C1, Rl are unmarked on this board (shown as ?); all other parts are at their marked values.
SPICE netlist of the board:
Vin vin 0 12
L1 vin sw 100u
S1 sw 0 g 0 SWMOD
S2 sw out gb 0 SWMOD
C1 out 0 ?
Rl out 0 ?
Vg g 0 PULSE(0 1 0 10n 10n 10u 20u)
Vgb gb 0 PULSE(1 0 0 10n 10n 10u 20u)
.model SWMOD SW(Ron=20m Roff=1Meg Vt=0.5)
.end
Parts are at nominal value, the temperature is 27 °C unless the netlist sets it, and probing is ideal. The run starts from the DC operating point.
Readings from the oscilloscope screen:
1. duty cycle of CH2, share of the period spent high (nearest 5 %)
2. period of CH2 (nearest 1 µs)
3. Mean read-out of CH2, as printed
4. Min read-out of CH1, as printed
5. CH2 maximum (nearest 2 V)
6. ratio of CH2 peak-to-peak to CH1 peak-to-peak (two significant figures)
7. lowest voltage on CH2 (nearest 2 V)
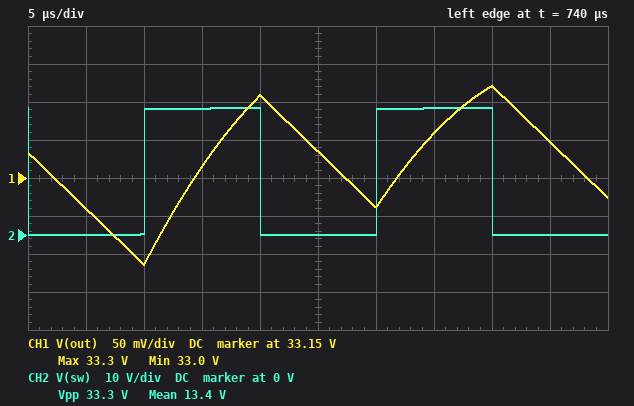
50 %
20 µs
13.4 V
33.0 V
34 V
140
0 V
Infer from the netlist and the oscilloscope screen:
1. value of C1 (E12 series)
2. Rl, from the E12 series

150 µF
15 Ω
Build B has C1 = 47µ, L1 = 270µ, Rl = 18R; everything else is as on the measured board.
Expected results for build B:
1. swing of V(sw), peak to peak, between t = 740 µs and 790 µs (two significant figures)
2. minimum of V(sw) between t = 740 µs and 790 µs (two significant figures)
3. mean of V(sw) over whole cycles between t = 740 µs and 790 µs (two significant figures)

32 V
53 mV
16 V
